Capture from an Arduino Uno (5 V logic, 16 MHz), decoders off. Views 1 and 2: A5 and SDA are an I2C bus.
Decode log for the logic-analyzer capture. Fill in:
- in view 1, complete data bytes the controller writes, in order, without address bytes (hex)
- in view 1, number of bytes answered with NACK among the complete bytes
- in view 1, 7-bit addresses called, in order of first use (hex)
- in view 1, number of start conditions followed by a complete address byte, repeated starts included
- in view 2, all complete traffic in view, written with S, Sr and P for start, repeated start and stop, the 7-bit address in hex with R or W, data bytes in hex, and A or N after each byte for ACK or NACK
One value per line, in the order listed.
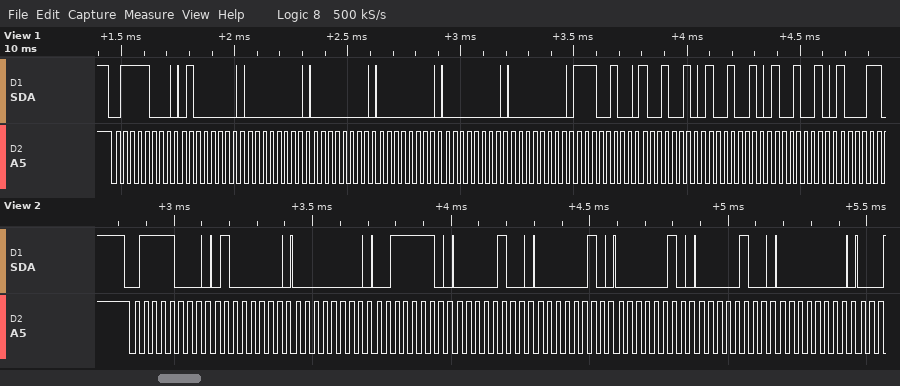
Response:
40 00 00 00 00 00 E4 92 92 92
0
0x3C
1
S 3CW A 40 A 00 A 3E A 04 A 02 A 02 A 04 A 00 A
